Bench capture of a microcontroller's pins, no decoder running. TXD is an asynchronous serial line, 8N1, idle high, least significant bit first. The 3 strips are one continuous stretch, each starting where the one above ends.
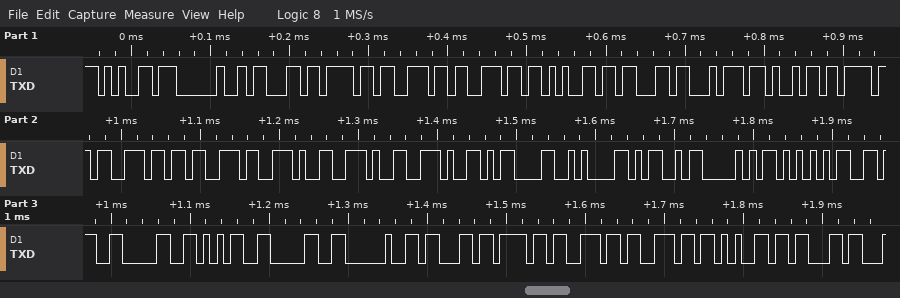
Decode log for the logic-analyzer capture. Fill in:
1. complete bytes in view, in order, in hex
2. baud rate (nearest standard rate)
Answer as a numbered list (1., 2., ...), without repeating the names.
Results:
1. 0x65 0x20 0x63 0x6F 0x6E 0x6E 0x65 0x63 0x74 0x69 0x6F 0x6E 0x73 0x2E 0x2E 0x2E 0x0D 0x0A 0x4D 0x50 0x55 0x36 0x30 0x35 0x30 0x20 0x63 0x6F 0x6E 0x6E 0x65 0x63
2. 115200 baud
